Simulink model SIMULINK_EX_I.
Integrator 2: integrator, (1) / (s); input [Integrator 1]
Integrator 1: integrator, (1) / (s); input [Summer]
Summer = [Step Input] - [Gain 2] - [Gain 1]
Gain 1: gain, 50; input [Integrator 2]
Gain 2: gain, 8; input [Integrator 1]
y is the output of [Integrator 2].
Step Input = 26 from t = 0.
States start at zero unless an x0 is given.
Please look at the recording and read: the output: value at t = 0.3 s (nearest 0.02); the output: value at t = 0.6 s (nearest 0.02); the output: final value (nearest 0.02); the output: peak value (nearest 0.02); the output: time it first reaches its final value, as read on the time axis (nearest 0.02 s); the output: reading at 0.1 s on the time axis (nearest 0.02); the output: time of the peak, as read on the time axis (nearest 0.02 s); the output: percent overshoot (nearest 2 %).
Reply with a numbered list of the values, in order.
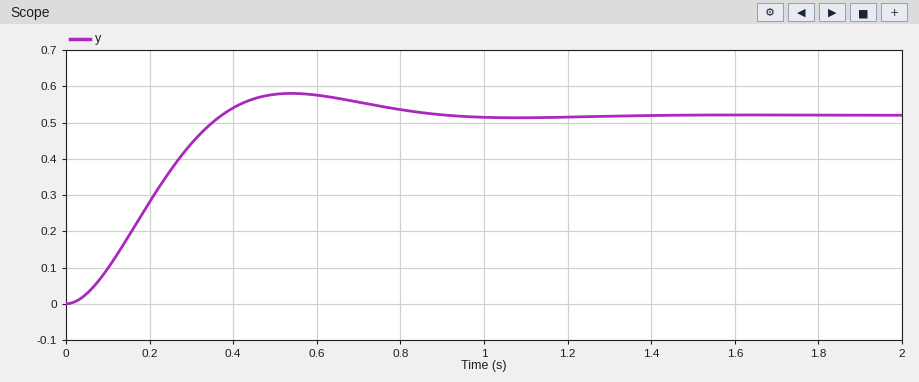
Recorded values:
1. 0.44
2. 0.58
3. 0.52
4. 0.58
5. 0.38 s
6. 0.10
7. 0.54 s
8. 12 %
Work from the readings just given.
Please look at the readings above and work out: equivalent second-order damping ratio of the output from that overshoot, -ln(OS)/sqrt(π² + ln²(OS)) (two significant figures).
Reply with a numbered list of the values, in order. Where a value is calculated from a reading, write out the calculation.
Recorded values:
1. ln(0.12) = -2.120; 2.120 / sqrt(9.870 + 4.496) = 0.56
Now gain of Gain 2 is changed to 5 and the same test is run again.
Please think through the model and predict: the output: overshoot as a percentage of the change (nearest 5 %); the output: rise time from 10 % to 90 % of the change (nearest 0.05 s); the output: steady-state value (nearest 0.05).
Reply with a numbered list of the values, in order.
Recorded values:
1. 30 %
2. 0.20 s
3. 0.50
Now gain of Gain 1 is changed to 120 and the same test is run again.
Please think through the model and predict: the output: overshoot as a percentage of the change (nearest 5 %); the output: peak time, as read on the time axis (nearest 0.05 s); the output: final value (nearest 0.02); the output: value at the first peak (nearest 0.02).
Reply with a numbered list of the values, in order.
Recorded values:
1. 30 %
2. 0.30 s
3. 0.22
4. 0.28
